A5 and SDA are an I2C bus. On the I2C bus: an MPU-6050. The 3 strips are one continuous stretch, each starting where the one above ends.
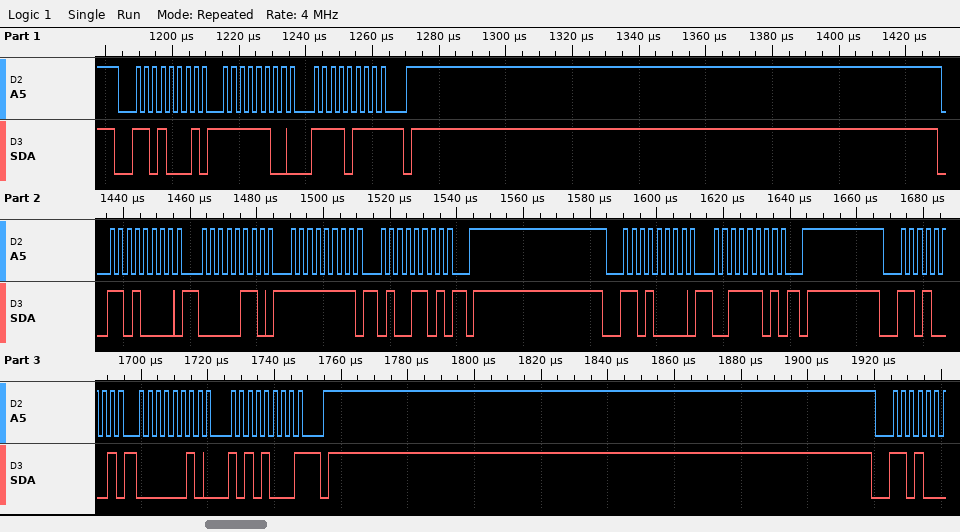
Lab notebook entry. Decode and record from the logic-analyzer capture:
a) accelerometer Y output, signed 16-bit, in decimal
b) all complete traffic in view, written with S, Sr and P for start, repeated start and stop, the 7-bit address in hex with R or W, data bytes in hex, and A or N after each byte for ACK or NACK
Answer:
680
S 68R A FC A F7 N P S 68W A 06 A FF A 4D A P S 68W A 3D A P S 68R A 02 A A8 N P
